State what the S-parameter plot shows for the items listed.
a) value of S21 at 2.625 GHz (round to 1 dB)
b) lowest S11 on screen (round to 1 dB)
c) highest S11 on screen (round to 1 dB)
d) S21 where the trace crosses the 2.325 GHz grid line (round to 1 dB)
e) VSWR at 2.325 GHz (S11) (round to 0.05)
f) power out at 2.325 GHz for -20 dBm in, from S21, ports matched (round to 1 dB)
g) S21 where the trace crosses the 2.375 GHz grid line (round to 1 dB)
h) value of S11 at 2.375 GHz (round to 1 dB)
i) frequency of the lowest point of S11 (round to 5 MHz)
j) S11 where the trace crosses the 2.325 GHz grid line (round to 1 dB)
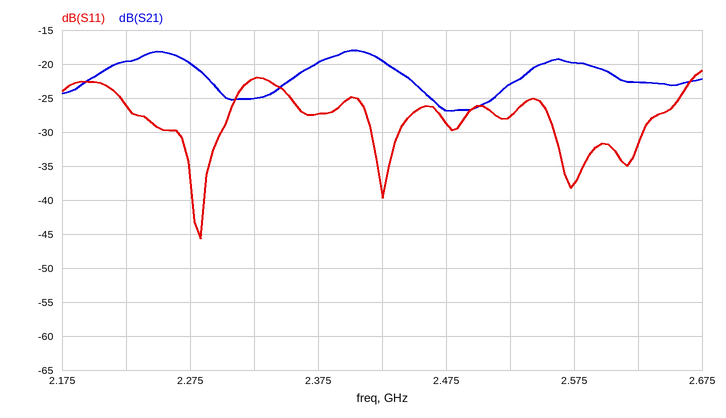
-23 dB
-46 dB
-21 dB
-25 dB
1.15
-45 dBm
-20 dB
-27 dB
2.285 GHz
-22 dB
